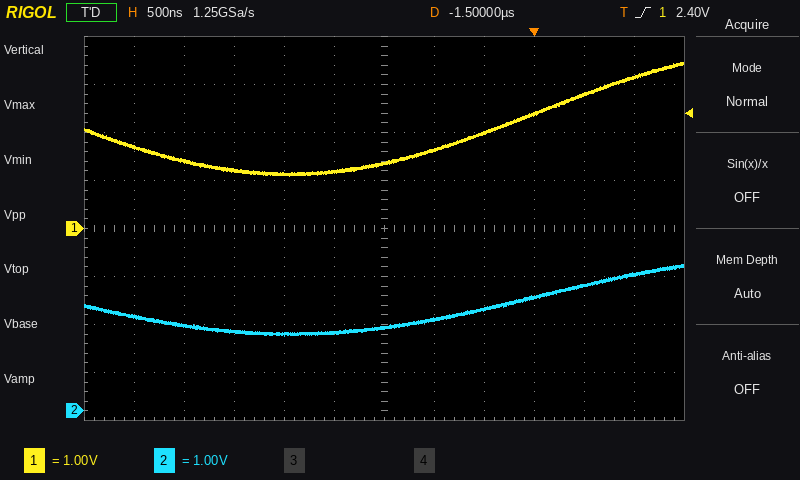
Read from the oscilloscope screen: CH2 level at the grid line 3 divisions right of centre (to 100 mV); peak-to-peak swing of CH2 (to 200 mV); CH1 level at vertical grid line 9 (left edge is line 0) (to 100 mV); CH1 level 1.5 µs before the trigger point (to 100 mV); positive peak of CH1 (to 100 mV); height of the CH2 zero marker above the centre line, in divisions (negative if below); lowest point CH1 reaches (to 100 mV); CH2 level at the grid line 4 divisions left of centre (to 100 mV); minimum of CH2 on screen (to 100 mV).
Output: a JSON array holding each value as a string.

["2.4 V", "1.4 V", "2.4 V", "1.4 V", "3.5 V", "-3.8 div", "1.1 V", "1.8 V", "1.6 V"]
